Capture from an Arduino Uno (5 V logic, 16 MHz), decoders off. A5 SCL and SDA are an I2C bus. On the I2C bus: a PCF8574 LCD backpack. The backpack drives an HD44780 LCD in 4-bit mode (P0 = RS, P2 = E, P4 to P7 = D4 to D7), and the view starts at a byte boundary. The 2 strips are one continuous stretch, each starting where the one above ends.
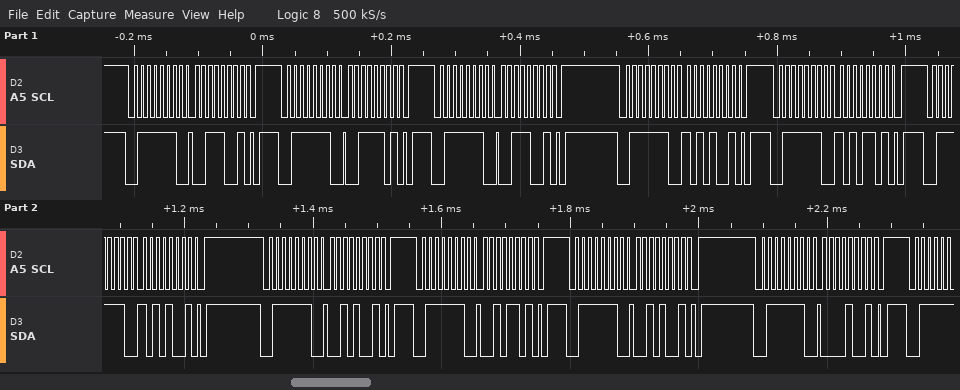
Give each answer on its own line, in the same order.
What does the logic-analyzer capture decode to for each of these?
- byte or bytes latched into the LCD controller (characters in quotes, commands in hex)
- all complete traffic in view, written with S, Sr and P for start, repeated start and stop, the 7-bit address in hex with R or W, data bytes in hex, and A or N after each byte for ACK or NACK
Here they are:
':'
S 3FW A 39 A P S 3FW A 3D A P S 3FW A 39 A P S 3FW A A9 A P S 3FW A AD A P S 3FW A A9 A P S 3FW A 29 A P S 3FW A 2D A P S 3FW A 29 A P S 3FW A 09 A P
